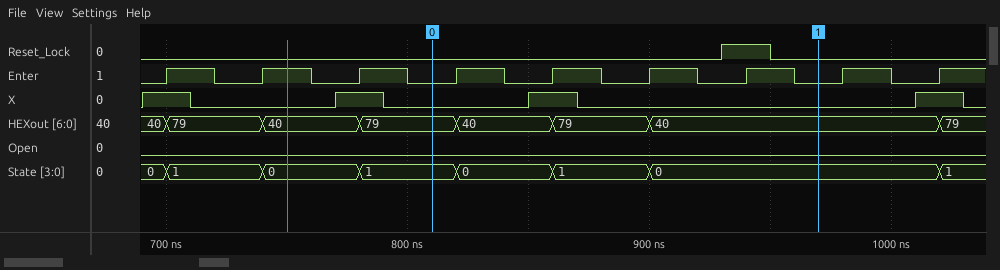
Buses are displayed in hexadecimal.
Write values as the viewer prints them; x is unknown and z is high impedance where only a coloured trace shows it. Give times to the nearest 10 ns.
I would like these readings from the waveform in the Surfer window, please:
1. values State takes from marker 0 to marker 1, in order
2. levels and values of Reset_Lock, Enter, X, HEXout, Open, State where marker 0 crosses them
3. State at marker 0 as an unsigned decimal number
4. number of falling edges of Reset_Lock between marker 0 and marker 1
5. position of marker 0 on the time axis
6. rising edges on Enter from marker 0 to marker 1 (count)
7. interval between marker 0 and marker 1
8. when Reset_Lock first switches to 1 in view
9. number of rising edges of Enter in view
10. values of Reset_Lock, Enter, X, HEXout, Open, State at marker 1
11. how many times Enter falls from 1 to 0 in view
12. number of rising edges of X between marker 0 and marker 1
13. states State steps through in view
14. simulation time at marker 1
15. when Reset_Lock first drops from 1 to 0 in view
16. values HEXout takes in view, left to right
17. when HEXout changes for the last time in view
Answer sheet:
1, 0, 1, 0
Reset_Lock=0, Enter=0, X=0, HEXout=79, Open=0, State=1
1
1
810 ns
4
160 ns
930 ns
9
Reset_Lock=0, Enter=0, X=0, HEXout=40, Open=0, State=0
8
1
0, 1, 0, 1, 0, 1, 0, 1
970 ns
950 ns
40, 79, 40, 79, 40, 79, 40, 79
1020 ns
